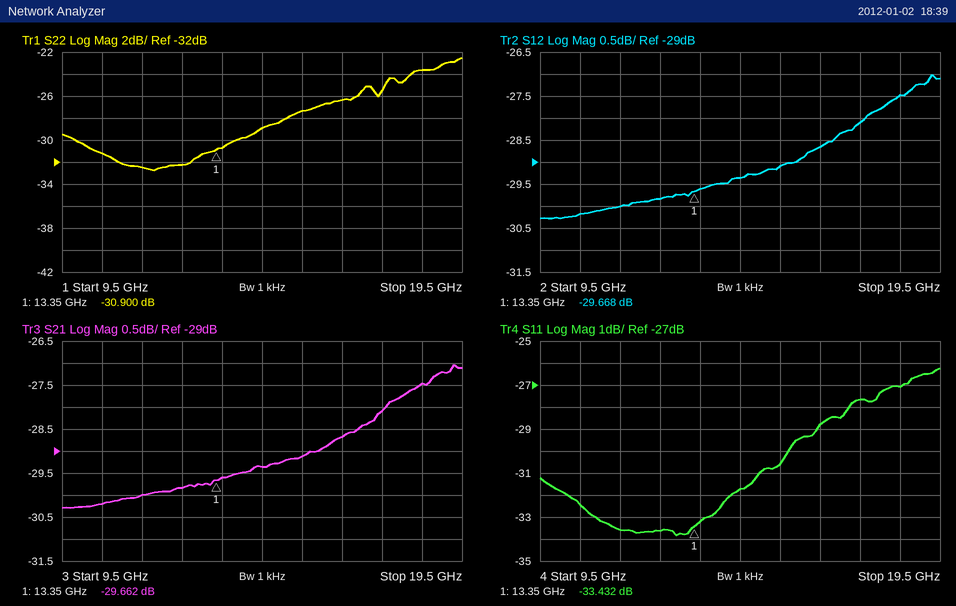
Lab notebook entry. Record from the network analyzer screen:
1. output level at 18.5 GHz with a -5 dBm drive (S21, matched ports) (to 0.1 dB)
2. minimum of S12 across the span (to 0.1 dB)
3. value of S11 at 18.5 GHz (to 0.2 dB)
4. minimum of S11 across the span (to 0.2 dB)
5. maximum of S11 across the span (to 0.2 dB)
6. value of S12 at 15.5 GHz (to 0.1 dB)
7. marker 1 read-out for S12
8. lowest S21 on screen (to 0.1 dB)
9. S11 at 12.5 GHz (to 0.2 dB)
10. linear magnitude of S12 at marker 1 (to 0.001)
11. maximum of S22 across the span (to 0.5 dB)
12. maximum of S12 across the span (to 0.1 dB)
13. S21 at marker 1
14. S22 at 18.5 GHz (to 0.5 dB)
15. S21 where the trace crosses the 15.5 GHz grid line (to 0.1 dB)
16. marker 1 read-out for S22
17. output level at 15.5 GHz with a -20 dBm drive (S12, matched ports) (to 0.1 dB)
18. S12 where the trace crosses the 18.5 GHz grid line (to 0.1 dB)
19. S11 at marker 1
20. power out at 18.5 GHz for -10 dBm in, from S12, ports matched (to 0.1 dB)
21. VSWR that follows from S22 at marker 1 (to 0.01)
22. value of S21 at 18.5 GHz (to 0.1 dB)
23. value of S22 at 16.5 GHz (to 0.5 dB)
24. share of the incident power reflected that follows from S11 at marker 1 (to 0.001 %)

-32.5 dBm
-30.3 dB
-27.0 dB
-33.8 dB
-26.2 dB
-29.1 dB
-29.668 dB
-30.3 dB
-33.6 dB
0.033
-22.5 dB
-27.0 dB
-29.662 dB
-23.5 dB
-29.1 dB
-30.900 dB
-49.1 dBm
-27.5 dB
-33.432 dB
-37.5 dBm
1.06
-27.5 dB
-26.5 dB
0.045 %
